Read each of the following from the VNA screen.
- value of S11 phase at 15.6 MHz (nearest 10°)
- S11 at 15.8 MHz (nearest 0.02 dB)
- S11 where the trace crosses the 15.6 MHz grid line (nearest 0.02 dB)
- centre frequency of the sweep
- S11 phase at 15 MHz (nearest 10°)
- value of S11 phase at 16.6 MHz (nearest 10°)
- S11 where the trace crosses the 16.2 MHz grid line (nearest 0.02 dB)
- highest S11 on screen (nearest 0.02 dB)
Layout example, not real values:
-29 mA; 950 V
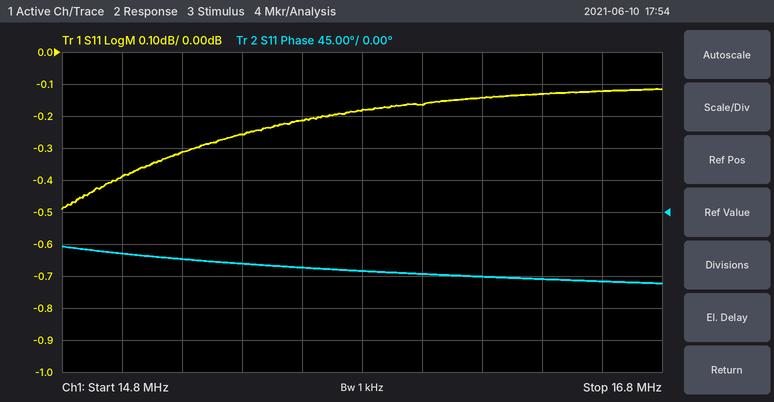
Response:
-80°; -0.18 dB; -0.22 dB; 15.8 MHz; -60°; -100°; -0.14 dB; -0.12 dB
